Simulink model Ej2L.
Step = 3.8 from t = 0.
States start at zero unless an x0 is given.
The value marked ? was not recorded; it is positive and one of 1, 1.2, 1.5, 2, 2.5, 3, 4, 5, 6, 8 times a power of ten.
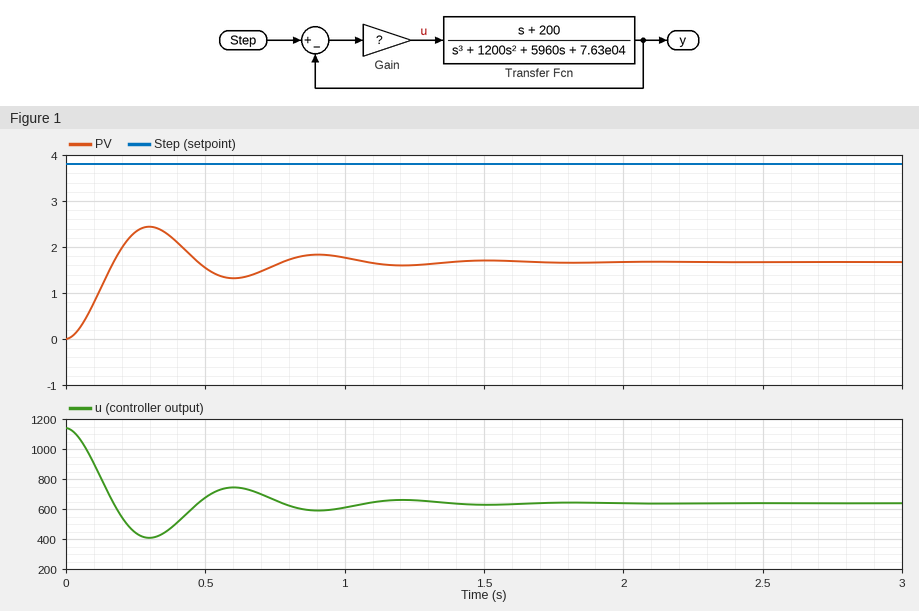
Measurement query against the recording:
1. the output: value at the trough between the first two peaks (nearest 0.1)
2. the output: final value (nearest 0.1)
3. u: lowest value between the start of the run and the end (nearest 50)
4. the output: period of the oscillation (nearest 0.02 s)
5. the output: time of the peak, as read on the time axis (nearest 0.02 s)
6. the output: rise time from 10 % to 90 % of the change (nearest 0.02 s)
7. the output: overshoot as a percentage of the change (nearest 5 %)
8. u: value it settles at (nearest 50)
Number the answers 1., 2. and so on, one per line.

1. 1.3
2. 1.7
3. 400
4. 0.60 s
5. 0.30 s
6. 0.12 s
7. 45 %
8. 650
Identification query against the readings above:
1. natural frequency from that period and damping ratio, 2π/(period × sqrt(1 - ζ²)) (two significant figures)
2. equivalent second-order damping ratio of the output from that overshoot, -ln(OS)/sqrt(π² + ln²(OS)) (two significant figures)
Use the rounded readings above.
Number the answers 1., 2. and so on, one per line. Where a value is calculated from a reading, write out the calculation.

1. 2π / (0.6 × sqrt(1 - 0.25²)) = 11 rad/s
2. ln(0.45) = -0.799; 0.799 / sqrt(9.870 + 0.638) = 0.25
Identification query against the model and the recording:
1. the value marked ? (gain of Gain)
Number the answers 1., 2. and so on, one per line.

1. 300
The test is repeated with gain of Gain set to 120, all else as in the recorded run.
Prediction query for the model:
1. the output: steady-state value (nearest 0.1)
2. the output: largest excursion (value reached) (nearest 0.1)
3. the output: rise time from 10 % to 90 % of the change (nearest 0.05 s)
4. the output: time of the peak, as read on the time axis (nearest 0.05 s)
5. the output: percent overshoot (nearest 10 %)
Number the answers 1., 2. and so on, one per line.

1. 0.9
2. 1.3
3. 0.15 s
4. 0.35 s
5. 40 %
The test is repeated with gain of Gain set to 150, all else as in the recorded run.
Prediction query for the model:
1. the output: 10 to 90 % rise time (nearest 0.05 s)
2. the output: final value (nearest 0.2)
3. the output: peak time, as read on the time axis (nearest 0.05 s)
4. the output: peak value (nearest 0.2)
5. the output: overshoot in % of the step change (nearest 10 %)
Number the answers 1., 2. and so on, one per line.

1. 0.15 s
2. 1.0
3. 0.35 s
4. 1.6
5. 40 %
